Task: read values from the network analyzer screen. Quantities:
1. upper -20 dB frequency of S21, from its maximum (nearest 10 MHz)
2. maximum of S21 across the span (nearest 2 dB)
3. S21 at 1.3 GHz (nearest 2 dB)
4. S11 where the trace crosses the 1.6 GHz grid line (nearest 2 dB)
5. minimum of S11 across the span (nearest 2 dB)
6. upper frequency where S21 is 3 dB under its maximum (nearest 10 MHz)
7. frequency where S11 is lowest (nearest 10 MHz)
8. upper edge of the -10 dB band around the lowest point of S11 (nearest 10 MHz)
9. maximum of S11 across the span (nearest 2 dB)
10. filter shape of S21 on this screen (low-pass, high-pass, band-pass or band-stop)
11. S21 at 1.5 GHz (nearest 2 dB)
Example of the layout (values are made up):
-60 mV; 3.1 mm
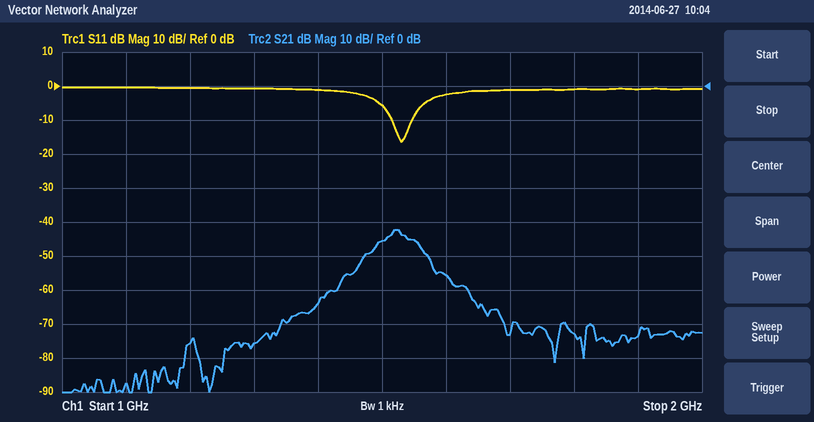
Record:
1.64 GHz; -42 dB; -76 dB; -2 dB; -16 dB; 1.55 GHz; 1.53 GHz; 1.55 GHz; 0 dB; band-pass; -46 dB
